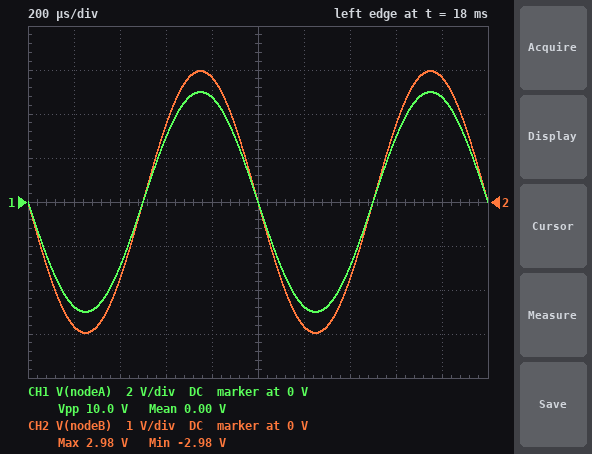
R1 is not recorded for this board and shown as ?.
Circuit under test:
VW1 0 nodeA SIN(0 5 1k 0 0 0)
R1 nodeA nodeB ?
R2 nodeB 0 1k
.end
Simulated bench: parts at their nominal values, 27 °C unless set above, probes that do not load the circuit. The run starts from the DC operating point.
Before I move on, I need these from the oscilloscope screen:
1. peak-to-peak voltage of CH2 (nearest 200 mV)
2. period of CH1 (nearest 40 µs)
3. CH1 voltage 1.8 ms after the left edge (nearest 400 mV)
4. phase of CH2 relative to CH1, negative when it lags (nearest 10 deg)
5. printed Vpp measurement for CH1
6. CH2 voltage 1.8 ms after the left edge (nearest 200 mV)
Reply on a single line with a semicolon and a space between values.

6.0 V; 1.00 ms; 4.8 V; 0 deg; 10.0 V; 2.8 V
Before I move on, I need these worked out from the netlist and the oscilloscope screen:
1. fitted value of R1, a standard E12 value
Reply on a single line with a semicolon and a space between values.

680 Ω
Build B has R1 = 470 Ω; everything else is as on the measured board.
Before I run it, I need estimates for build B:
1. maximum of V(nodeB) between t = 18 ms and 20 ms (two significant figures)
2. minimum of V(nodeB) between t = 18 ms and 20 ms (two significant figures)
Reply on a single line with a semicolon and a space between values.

3.4 V; -3.4 V
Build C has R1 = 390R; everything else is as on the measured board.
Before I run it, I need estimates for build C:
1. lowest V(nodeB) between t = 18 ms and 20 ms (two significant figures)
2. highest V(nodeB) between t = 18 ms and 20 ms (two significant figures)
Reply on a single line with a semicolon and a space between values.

-3.6 V; 3.6 V
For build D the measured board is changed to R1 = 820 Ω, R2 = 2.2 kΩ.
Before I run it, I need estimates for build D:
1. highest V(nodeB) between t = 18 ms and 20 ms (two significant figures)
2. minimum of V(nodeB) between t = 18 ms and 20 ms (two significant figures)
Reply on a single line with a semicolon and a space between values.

3.6 V; -3.6 V
